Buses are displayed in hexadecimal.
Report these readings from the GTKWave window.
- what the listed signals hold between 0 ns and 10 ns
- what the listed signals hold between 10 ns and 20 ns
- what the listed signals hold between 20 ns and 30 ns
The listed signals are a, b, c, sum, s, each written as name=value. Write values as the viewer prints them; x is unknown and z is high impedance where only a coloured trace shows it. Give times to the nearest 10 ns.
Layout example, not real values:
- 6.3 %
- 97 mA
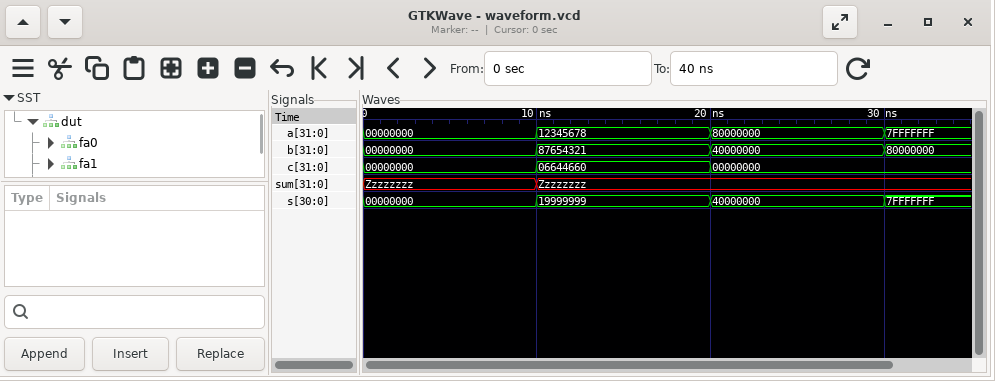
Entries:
- a=00000000, b=00000000, c=00000000, sum=Zzzzzzzz, s=00000000
- a=12345678, b=87654321, c=06644660, sum=Zzzzzzzz, s=19999999
- a=80000000, b=40000000, c=00000000, sum=Zzzzzzzz, s=40000000
